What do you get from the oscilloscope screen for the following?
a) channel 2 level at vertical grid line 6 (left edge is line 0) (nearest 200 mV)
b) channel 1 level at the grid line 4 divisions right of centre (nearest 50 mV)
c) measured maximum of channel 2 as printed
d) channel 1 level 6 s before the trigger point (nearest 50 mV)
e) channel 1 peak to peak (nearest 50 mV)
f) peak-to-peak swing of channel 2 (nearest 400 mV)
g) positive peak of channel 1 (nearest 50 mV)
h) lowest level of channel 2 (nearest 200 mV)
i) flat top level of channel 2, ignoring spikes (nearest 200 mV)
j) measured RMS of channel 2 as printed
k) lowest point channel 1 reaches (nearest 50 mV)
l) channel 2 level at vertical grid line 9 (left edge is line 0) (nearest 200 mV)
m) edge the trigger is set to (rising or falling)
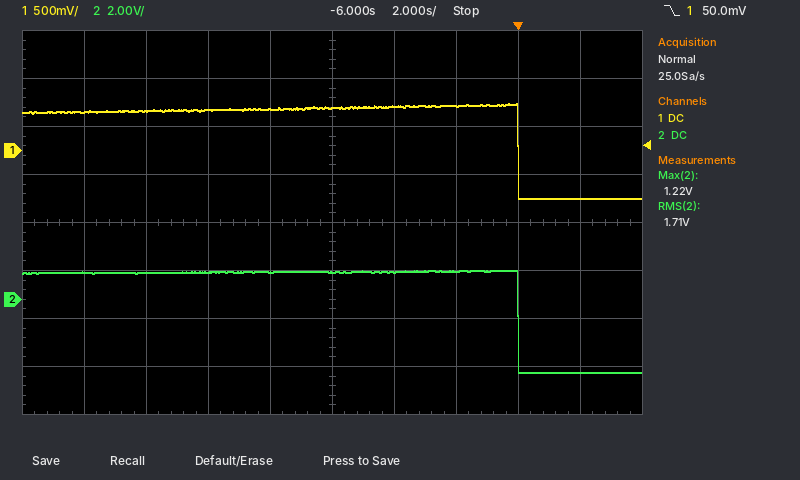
1.2 V
-500 mV
1.22 V
450 mV
1.00 V
4.4 V
500 mV
-3.0 V
1.2 V
1.71 V
-500 mV
-3.0 V
falling
